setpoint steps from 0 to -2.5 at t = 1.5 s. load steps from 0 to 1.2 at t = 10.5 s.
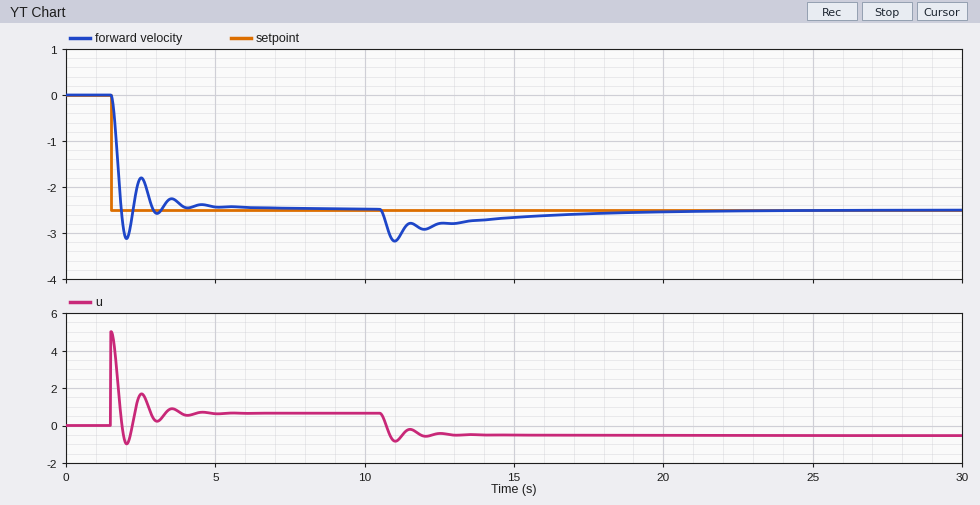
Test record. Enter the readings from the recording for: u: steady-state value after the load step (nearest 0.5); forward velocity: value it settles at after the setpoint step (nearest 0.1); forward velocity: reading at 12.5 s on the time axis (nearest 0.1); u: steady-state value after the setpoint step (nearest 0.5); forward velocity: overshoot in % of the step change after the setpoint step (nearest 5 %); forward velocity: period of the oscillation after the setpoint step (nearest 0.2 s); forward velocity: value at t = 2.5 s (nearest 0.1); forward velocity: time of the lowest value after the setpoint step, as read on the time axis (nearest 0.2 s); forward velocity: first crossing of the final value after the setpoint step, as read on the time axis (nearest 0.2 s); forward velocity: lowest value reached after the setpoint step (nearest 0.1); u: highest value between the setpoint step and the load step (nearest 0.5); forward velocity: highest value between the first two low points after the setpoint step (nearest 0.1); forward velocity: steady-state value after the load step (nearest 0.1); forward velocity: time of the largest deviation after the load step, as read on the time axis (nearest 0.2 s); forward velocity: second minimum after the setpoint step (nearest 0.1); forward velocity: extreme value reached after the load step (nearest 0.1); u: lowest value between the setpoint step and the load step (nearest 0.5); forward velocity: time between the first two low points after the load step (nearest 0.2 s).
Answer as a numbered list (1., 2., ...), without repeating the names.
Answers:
1. -0.5
2. -2.5
3. -2.8
4. 0.5
5. 25 %
6. 1.0 s
7. -1.8
8. 2.0 s
9. 1.8 s
10. -3.1
11. 5.0
12. -1.8
13. -2.5
14. 11.0 s
15. -2.6
16. -3.2
17. -1.0
18. 1.0 s
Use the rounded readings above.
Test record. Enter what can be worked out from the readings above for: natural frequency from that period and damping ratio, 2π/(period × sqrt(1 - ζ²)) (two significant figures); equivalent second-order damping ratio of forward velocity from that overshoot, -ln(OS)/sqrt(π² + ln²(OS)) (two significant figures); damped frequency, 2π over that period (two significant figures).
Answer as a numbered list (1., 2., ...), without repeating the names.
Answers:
1. 6.9 rad/s
2. 0.40
3. 6.3 rad/s
